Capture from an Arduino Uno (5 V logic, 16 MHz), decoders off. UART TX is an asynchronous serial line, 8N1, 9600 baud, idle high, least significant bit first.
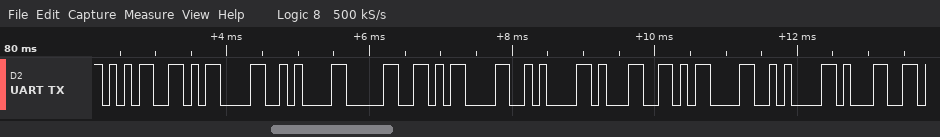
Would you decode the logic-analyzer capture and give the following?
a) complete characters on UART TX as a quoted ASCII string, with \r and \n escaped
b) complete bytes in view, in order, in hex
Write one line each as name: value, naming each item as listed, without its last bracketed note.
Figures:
complete characters on UART TX as a quoted ASCII string, with \r and \n escaped: "5\r\n0\r\n1\r\n1"
complete bytes in view, in order, in hex: 0x35 0x0D 0x0A 0x30 0x0D 0x0A 0x31 0x0D 0x0A 0x31
